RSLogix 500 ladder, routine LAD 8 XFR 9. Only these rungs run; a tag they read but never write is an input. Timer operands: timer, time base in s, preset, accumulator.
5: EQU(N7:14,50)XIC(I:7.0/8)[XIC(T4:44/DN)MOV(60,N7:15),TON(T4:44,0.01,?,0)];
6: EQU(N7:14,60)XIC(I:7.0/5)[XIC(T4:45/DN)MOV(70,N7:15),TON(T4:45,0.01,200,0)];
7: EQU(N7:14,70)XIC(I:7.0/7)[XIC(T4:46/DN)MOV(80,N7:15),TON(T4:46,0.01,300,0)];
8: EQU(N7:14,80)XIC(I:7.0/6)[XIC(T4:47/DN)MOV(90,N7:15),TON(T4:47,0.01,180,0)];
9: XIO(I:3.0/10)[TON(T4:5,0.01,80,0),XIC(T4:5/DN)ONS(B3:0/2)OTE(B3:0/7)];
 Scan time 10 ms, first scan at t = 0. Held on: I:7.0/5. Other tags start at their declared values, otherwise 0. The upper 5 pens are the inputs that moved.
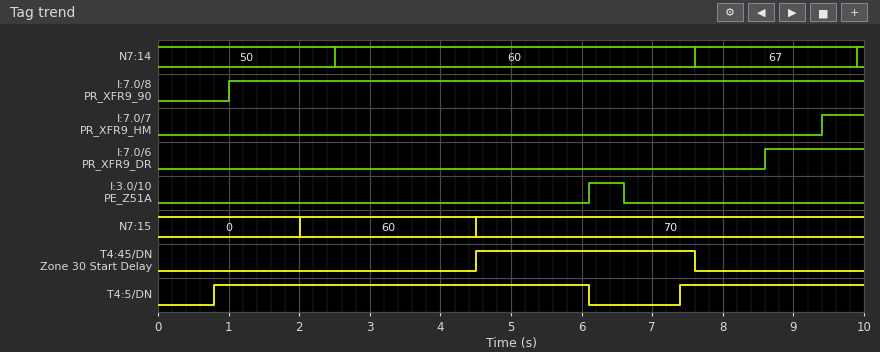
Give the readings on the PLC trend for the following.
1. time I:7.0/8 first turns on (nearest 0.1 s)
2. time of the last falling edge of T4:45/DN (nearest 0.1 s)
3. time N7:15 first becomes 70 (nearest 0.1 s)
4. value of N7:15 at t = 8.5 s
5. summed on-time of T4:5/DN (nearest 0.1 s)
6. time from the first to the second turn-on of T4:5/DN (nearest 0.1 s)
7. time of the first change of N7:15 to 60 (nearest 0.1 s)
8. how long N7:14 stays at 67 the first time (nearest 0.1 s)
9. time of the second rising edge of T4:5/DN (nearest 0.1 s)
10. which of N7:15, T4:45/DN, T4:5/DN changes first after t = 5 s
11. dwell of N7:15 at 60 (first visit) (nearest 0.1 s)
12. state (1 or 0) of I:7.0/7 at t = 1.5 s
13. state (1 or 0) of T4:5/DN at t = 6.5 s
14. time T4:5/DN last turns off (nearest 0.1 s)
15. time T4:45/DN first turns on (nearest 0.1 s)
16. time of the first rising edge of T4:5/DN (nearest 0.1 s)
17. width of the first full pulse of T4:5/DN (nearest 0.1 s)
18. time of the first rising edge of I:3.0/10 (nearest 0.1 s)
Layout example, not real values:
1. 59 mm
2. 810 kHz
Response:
1. 1.0 s
2. 7.6 s
3. 4.5 s
4. 70
5. 7.9 s
6. 6.6 s
7. 2.0 s
8. 2.3 s
9. 7.4 s
10. T4:5/DN
11. 2.5 s
12. 0
13. 0
14. 6.1 s
15. 4.5 s
16. 0.8 s
17. 5.3 s
18. 6.1 s
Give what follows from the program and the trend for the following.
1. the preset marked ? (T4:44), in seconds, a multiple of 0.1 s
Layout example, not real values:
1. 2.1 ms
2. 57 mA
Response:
1. 1.0 s
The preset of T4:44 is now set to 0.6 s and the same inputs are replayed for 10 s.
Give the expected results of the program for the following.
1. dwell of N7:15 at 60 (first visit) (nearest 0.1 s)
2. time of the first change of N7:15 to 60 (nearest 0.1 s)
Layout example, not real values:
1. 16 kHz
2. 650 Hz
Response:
1. 2.9 s
2. 1.6 s
